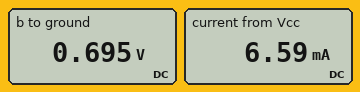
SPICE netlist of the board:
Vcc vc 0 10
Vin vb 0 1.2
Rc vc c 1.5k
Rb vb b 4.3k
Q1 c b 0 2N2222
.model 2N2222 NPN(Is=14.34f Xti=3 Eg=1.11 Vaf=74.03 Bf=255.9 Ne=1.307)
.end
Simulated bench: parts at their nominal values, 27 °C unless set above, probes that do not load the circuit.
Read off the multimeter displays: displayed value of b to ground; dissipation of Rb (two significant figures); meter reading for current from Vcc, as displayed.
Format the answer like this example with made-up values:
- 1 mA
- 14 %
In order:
- 0.695 V
- 59 µW
- 6.59 mA
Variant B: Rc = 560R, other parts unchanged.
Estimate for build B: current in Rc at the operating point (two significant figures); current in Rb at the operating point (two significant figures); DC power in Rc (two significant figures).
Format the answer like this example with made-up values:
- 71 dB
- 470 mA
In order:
- 18 mA
- 110 µA
- 170 mW
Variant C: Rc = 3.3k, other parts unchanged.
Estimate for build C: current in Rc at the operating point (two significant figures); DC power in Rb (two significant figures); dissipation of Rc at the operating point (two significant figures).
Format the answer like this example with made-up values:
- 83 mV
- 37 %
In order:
- 3.0 mA
- 64 µW
- 30 mW
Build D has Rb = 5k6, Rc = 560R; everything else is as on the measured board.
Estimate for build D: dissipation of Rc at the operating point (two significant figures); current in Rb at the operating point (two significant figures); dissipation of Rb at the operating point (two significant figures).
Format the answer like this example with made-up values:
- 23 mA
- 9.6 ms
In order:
- 170 mW
- 86 µA
- 41 µW
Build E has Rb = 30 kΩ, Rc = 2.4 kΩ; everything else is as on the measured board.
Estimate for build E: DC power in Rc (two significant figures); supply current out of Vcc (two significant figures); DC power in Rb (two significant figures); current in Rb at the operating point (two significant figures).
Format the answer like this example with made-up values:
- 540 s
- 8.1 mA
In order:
- 40 mW
- 4.1 mA
- 8.9 µW
- 17 µA
